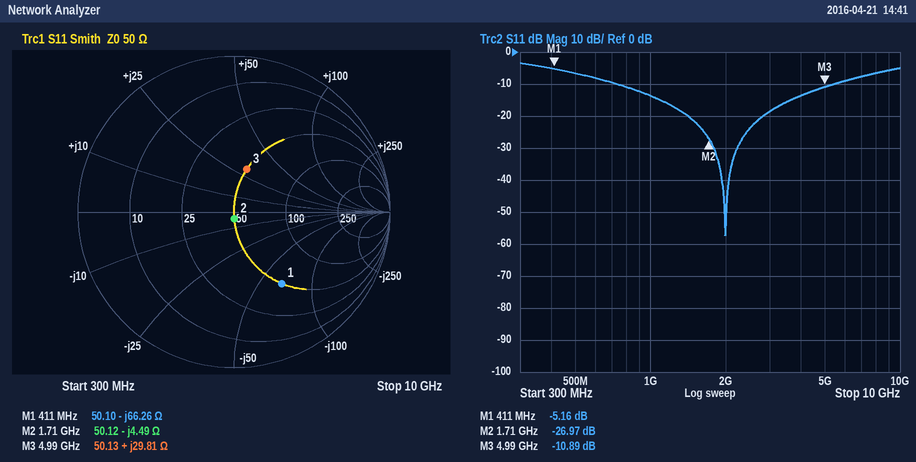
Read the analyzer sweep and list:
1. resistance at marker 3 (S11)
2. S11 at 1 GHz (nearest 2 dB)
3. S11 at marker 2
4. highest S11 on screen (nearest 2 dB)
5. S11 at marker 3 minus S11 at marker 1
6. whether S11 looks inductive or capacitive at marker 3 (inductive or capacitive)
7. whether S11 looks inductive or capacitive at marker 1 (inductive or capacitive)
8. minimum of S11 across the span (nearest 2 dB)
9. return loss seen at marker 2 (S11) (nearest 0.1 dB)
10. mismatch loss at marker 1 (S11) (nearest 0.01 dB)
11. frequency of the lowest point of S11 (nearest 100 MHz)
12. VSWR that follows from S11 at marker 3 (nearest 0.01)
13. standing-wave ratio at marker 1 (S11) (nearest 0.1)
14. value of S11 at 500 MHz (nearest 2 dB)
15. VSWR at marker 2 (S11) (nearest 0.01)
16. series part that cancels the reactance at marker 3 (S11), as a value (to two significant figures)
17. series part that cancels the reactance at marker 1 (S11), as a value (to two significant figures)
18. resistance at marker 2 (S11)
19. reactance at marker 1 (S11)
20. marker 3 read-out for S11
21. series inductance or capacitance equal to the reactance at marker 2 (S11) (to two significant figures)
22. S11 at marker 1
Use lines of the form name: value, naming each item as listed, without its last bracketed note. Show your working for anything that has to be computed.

resistance at marker 3: 50.13 Ω
S11 at 1 GHz: -14 dB
S11 at marker 2: -26.97 dB
highest S11 on screen: -4 dB
S11 at marker 3 minus S11 at marker 1: -10.89 − (-5.16) = -5.73 dB
whether S11 looks inductive or capacitive at marker 3: inductive
whether S11 looks inductive or capacitive at marker 1: capacitive
minimum of S11 across the span: -58 dB
return loss seen at marker 2 (S11): 27.0 dB
mismatch loss at marker 1 (S11): −10 log10(1 − 10^(-5.16/10)) ≈ 1.58 dB
frequency of the lowest point of S11: 2.0 GHz
VSWR that follows from S11 at marker 3: (1 + 0.2854)/(1 − 0.2854) ≈ 1.80
standing-wave ratio at marker 1 (S11): 3.5
value of S11 at 500 MHz: -6 dB
VSWR at marker 2 (S11): (1 + 0.0448)/(1 − 0.0448) ≈ 1.09
series part that cancels the reactance at marker 3 (S11), as a value: C = 1/(2π × 4.99 GHz × 29.81 Ω) ≈ 1.1 pF
series part that cancels the reactance at marker 1 (S11), as a value: L = 66.26 Ω/(2π × 411 MHz) ≈ 26 nH
resistance at marker 2: 50.12 Ω
reactance at marker 1: -66.26 Ω
marker 3 read-out for S11: -10.89 dB
series inductance or capacitance equal to the reactance at marker 2 (S11): C = 1/(2π × 1.71 GHz × 4.49 Ω) ≈ 21 pF
S11 at marker 1: -5.16 dB
